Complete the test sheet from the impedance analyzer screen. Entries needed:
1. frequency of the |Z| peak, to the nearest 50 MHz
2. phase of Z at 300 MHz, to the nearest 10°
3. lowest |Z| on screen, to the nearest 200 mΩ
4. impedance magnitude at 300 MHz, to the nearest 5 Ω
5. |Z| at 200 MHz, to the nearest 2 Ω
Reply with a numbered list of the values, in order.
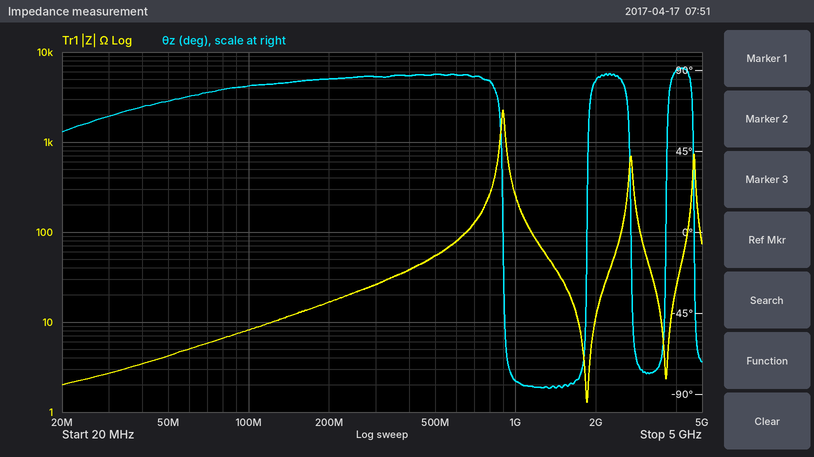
1. 900 MHz
2. 90°
3. 1.2 Ω
4. 25 Ω
5. 16 Ω
